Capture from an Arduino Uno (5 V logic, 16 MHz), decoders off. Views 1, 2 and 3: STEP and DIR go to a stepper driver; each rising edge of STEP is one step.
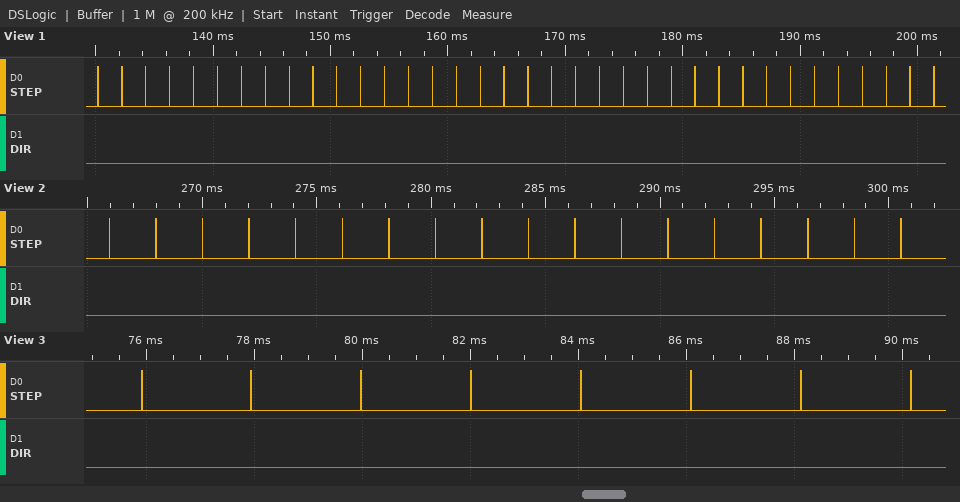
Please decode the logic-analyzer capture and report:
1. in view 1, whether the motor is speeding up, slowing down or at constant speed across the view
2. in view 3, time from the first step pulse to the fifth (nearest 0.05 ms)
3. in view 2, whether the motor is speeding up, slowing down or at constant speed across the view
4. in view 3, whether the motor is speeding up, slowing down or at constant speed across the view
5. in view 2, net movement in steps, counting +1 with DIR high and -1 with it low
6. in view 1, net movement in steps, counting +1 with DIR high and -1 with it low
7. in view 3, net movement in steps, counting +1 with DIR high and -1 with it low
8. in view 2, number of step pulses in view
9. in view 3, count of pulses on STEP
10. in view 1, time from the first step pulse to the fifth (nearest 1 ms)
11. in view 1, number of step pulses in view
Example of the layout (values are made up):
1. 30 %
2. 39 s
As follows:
1. constant speed
2. 8.15 ms
3. constant speed
4. constant speed
5. -18
6. -36
7. -8
8. 18
9. 8
10. 8 ms
11. 36
